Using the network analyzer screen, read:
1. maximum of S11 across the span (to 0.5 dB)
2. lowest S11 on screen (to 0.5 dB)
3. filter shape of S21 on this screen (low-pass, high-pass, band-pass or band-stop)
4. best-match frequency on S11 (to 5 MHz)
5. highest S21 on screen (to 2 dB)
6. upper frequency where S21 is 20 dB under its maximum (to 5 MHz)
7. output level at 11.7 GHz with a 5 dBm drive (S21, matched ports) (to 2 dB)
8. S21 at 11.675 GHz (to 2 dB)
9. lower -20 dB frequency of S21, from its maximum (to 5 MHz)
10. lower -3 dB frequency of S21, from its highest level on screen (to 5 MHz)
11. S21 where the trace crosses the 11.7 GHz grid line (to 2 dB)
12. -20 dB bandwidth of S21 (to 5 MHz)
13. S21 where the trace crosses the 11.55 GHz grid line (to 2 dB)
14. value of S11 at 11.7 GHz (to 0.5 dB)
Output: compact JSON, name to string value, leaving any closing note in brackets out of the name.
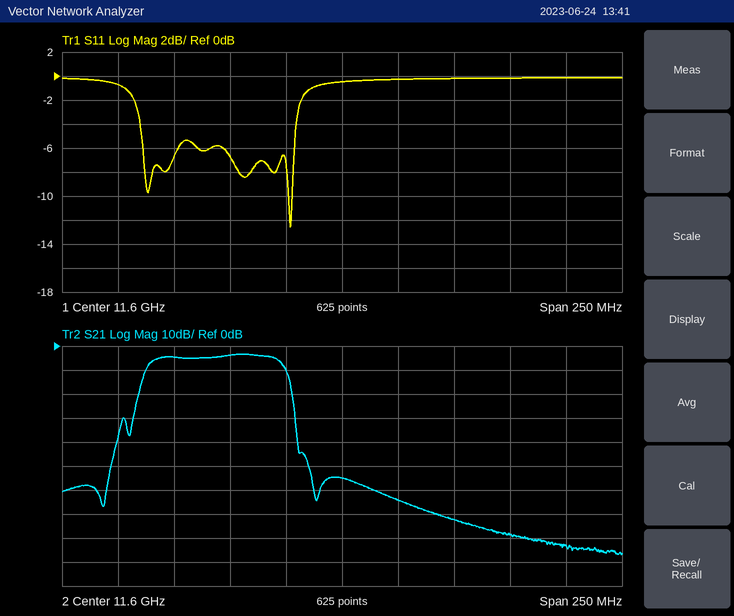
{"maximum of S11 across the span": "0.0 dB", "lowest S11 on screen": "-12.5 dB", "filter shape of S21 on this screen": "band-pass", "best-match frequency on S11": "11.575 GHz", "highest S21 on screen": "-4 dB", "upper frequency where S21 is 20 dB under its maximum": "11.580 GHz", "output level at 11.7 GHz with a 5 dBm drive (S21, matched ports)": "-78 dBm", "S21 at 11.675 GHz": "-78 dB", "lower -20 dB frequency of S21, from its maximum": "11.510 GHz", "lower -3 dB frequency of S21, from its highest level on screen": "11.515 GHz", "S21 where the trace crosses the 11.7 GHz grid line": "-84 dB", "-20 dB bandwidth of S21": "70 MHz", "S21 where the trace crosses the 11.55 GHz grid line": "-4 dB", "value of S11 at 11.7 GHz": "0.0 dB"}
